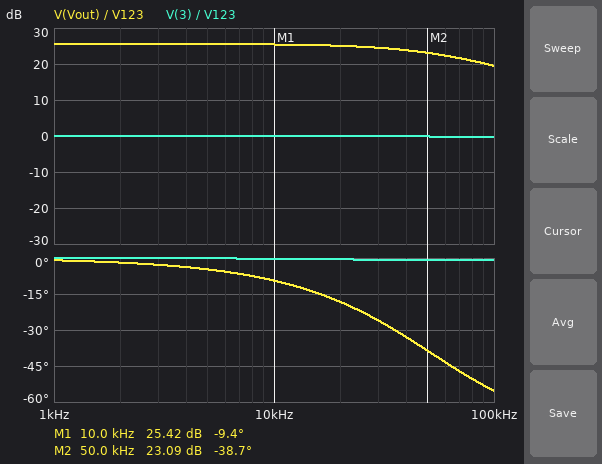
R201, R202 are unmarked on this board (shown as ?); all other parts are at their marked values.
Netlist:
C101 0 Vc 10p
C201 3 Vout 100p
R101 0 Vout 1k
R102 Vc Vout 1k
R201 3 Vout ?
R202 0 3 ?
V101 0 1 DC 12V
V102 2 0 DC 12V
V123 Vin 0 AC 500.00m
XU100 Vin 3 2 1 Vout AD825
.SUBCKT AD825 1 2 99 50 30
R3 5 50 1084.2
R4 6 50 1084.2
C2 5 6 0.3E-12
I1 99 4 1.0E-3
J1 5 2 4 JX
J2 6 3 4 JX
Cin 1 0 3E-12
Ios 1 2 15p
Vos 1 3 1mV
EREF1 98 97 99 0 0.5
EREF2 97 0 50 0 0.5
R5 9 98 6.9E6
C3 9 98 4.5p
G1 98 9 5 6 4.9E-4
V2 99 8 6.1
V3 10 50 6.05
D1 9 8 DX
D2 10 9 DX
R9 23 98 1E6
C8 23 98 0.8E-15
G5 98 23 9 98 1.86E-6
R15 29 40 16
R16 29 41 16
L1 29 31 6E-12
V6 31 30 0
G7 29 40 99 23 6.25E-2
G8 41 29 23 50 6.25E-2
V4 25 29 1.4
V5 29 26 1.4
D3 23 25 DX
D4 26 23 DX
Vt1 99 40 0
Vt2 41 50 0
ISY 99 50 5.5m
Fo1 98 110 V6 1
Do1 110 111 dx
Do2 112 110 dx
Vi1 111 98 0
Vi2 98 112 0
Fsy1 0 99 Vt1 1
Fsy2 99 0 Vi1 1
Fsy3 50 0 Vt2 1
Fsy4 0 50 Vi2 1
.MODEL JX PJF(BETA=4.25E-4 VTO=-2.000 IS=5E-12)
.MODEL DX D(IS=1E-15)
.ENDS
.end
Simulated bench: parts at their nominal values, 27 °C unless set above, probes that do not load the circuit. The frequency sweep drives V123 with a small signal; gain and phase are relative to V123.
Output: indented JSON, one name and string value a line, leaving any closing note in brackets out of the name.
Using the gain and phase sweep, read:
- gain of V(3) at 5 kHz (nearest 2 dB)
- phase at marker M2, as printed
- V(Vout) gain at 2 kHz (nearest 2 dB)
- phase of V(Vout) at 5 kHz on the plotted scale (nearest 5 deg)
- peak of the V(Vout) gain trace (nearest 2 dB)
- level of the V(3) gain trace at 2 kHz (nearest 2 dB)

{
  "gain of V(3) at 5 kHz": "0 dB",
  "phase at marker M2, as printed": "-38.7 deg",
  "V(Vout) gain at 2 kHz": "26 dB",
  "phase of V(Vout) at 5 kHz on the plotted scale": "-5 deg",
  "peak of the V(Vout) gain trace": "26 dB",
  "level of the V(3) gain trace at 2 kHz": "0 dB"
}
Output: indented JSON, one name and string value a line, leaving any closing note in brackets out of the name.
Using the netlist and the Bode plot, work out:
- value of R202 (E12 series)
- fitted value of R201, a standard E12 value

{
  "value of R202": "1.5 kΩ",
  "fitted value of R201, a standard E12 value": "27 kΩ"
}
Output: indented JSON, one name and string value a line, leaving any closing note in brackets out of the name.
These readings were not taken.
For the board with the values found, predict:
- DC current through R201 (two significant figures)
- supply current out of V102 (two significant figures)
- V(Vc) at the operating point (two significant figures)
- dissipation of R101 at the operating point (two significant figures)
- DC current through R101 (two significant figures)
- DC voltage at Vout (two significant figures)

{
  "DC current through R201": "660 nA",
  "supply current out of V102": "6.5 mA",
  "V(Vc) at the operating point": "-19 mV",
  "dissipation of R101 at the operating point": "360 nW",
  "DC current through R101": "19 µA",
  "DC voltage at Vout": "-19 mV"
}
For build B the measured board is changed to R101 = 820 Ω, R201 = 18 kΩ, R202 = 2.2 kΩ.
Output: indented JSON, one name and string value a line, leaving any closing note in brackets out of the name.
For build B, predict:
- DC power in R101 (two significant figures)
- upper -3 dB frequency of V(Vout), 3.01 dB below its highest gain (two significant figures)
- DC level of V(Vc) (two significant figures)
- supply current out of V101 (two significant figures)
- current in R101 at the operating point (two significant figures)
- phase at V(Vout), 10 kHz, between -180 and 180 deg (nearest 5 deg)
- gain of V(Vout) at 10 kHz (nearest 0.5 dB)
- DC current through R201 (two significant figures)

{
  "DC power in R101": "100 nW",
  "upper -3 dB frequency of V(Vout), 3.01 dB below its highest gain": "88 kHz",
  "DC level of V(Vc)": "-9.2 mV",
  "supply current out of V101": "6.5 mA",
  "current in R101 at the operating point": "11 µA",
  "phase at V(Vout), 10 kHz, between -180 and 180 deg": "-5 deg",
  "gain of V(Vout) at 10 kHz": "19.0 dB",
  "DC current through R201": "450 nA"
}
